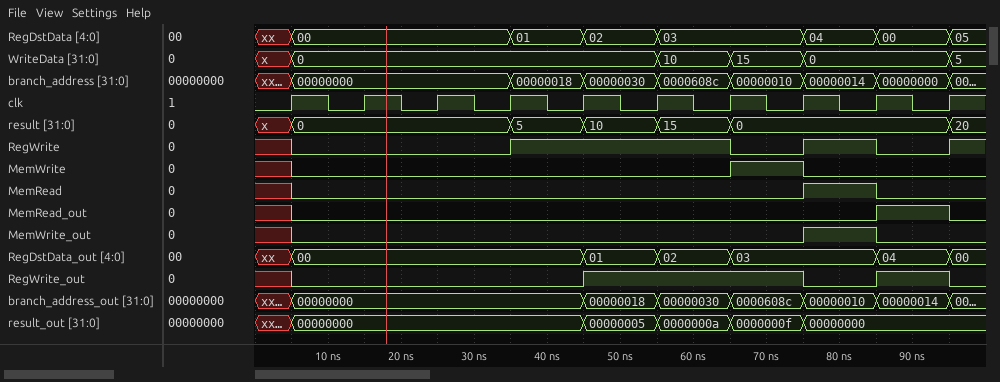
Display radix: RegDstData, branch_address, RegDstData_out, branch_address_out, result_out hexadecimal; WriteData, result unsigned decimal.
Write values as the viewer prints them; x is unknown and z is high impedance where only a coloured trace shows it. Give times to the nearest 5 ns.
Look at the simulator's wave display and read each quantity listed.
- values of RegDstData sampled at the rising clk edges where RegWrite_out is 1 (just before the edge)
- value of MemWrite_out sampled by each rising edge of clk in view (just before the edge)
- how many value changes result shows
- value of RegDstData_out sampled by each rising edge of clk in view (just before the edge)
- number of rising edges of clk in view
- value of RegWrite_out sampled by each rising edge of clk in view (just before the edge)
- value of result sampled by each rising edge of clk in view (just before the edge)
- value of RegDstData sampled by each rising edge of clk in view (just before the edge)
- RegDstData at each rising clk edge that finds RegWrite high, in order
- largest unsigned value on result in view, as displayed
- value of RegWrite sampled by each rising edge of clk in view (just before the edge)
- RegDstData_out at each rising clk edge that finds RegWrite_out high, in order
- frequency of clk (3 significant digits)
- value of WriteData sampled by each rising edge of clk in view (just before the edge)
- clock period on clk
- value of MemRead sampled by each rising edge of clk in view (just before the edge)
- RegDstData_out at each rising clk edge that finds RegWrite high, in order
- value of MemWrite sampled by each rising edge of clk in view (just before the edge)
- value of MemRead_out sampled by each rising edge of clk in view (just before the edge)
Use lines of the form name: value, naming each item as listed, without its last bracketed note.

values of RegDstData sampled at the rising clk edges where RegWrite_out is 1: 02, 03, 03, 00
value of MemWrite_out sampled by each rising edge of clk in view: x 0 0 0 0 0 0 0 1 0
how many value changes result shows: 6
value of RegDstData_out sampled by each rising edge of clk in view: xx, 00, 00, 00, 00, 01, 02, 03, 03, 04
number of rising edges of clk in view: 10
value of RegWrite_out sampled by each rising edge of clk in view: x 0 0 0 0 1 1 1 0 1
value of result sampled by each rising edge of clk in view: x, 0, 0, 0, 5, 10, 15, 0, 0, 0
value of RegDstData sampled by each rising edge of clk in view: xx, 00, 00, 00, 01, 02, 03, 03, 04, 00
RegDstData at each rising clk edge that finds RegWrite high, in order: 01, 02, 03, 04
largest unsigned value on result in view, as displayed: 20
value of RegWrite sampled by each rising edge of clk in view: x 0 0 0 1 1 1 0 1 0
RegDstData_out at each rising clk edge that finds RegWrite_out high, in order: 01, 02, 03, 04
frequency of clk: 100 MHz
value of WriteData sampled by each rising edge of clk in view: x, 0, 0, 0, 0, 0, 10, 15, 0, 0
clock period on clk: 10 ns
value of MemRead sampled by each rising edge of clk in view: x 0 0 0 0 0 0 0 1 0
RegDstData_out at each rising clk edge that finds RegWrite high, in order: 00, 01, 02, 03
value of MemWrite sampled by each rising edge of clk in view: x 0 0 0 0 0 0 1 0 0
value of MemRead_out sampled by each rising edge of clk in view: x 0 0 0 0 0 0 0 0 1
